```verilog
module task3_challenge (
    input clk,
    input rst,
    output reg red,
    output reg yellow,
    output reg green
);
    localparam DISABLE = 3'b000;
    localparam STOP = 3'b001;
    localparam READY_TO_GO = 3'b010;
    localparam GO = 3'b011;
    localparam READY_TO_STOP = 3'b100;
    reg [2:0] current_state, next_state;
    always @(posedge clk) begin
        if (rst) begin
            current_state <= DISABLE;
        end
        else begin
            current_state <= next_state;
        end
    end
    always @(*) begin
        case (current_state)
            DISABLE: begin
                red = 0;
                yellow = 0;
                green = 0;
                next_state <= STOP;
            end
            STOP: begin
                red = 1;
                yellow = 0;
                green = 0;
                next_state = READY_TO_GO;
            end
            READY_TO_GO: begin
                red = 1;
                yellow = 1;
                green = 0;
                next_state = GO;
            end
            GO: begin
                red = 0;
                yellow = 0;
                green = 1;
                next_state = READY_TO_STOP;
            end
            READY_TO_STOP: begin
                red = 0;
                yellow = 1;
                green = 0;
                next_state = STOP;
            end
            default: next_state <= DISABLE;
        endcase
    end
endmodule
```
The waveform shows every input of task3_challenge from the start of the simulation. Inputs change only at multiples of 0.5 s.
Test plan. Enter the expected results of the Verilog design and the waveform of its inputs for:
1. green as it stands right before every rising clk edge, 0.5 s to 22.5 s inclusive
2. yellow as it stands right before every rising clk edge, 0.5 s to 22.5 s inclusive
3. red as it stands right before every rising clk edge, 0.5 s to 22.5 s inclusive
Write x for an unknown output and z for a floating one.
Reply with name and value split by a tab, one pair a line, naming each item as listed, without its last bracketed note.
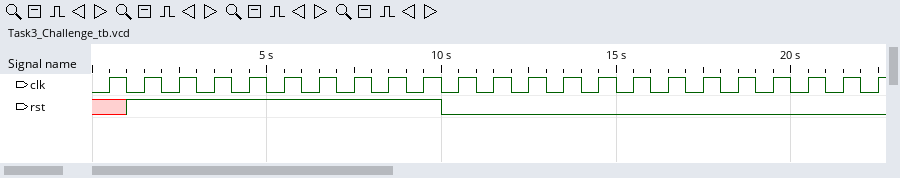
green as it stands right before every rising clk edge, 0.5 s to 22.5 s inclusive	x x 0 0 0 0 0 0 0 0 0 0 0 1 0 0 0 1 0 0 0 1 0
yellow as it stands right before every rising clk edge, 0.5 s to 22.5 s inclusive	x x 0 0 0 0 0 0 0 0 0 0 1 0 1 0 1 0 1 0 1 0 1
red as it stands right before every rising clk edge, 0.5 s to 22.5 s inclusive	x x 0 0 0 0 0 0 0 0 0 1 1 0 0 1 1 0 0 1 1 0 0
